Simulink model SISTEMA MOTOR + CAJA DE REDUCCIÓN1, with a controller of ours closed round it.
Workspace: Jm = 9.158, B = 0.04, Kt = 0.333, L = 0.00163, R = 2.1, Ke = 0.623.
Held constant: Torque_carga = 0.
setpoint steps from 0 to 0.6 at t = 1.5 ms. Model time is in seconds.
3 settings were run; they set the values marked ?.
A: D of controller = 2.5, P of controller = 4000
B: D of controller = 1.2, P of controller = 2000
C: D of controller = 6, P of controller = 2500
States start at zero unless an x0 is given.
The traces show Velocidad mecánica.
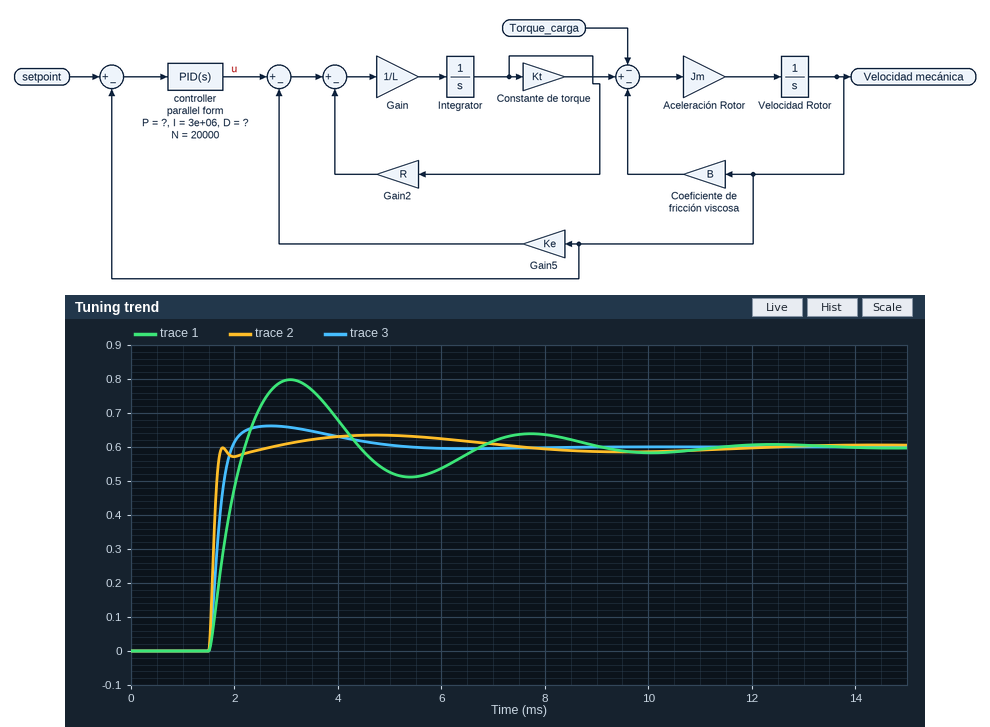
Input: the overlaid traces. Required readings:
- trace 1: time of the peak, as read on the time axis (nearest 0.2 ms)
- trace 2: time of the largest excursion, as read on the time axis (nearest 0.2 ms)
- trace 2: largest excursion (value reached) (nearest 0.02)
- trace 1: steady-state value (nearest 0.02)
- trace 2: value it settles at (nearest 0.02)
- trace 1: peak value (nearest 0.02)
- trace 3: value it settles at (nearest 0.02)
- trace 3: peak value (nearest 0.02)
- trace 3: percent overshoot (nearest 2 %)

3.0 ms
4.8 ms
0.64
0.60
0.60
0.80
0.60
0.66
10 %
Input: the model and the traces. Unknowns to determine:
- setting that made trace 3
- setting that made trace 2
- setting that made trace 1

A
C
B
